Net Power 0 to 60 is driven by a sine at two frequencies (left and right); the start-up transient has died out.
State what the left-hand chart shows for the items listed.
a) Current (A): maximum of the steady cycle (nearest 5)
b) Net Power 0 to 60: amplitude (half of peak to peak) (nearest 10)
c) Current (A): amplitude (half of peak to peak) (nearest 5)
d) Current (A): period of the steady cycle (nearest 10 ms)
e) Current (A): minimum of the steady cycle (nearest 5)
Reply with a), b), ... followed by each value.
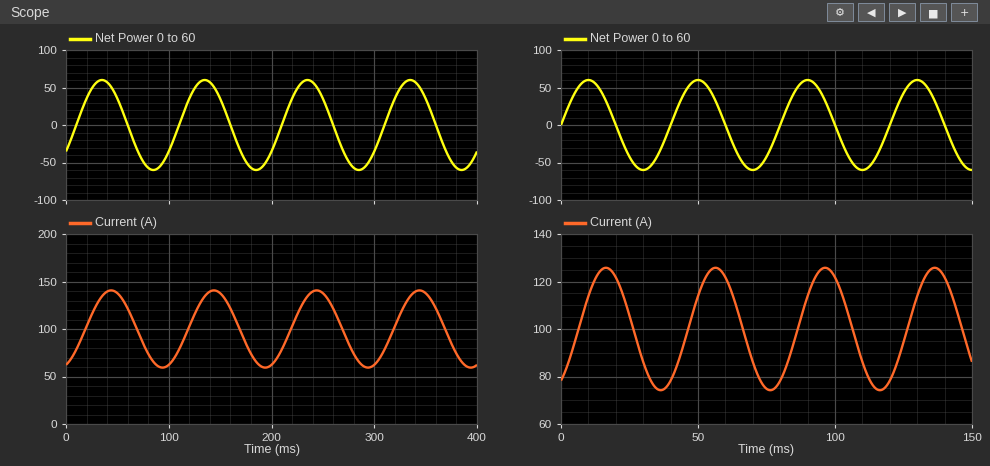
a) 140
b) 60
c) 40
d) 100 ms
e) 60
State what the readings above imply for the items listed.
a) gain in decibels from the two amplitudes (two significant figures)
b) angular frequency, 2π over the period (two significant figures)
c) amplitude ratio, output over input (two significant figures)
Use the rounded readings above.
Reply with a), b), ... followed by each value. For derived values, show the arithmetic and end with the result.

a) 20 log10(40 / 60) = -3.5 dB
b) 2π / 100 = 0.063 rad/ms
c) 40 / 60 = 0.67
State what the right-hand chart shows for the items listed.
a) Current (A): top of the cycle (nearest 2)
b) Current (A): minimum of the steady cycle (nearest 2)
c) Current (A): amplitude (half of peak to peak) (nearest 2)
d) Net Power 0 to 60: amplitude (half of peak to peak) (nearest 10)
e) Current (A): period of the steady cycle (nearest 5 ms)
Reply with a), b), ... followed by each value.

a) 126
b) 74
c) 26
d) 60
e) 40 ms
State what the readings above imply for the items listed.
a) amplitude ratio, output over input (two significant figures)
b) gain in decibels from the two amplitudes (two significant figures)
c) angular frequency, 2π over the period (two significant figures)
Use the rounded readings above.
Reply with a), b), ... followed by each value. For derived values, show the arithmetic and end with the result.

a) 26 / 60 = 0.43
b) 20 log10(26 / 60) = -7.3 dB
c) 2π / 40 = 0.16 rad/ms
